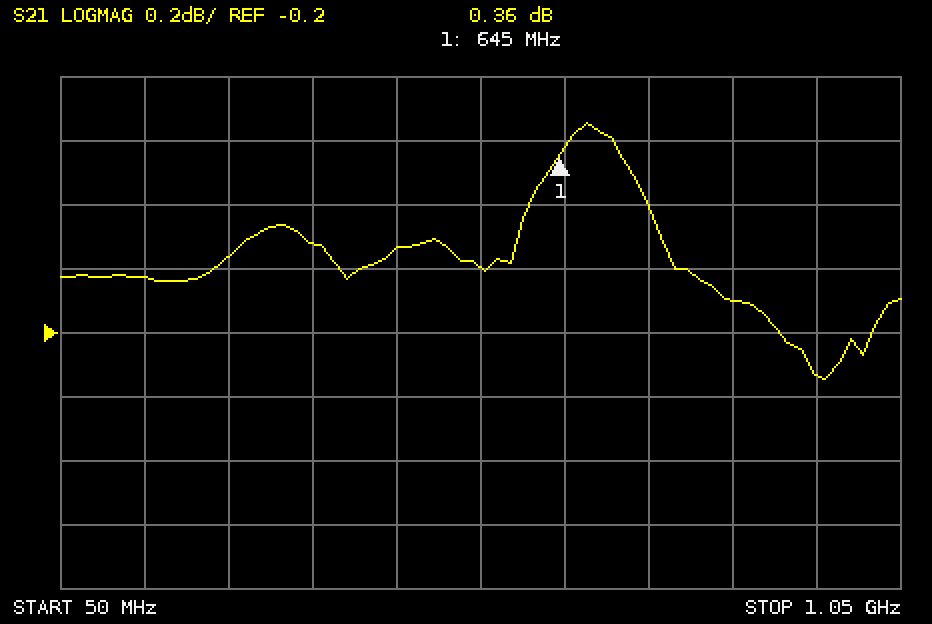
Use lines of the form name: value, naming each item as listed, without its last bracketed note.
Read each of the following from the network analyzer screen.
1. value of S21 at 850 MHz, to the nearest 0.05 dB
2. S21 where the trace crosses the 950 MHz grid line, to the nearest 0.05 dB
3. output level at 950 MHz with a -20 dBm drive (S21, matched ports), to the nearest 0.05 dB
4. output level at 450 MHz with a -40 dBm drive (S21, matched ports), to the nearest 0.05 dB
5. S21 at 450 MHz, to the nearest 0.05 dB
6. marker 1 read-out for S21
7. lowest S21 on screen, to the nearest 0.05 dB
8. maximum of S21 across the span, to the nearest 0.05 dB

value of S21 at 850 MHz, to the nearest 0.05 dB: -0.10 dB
S21 where the trace crosses the 950 MHz grid line, to the nearest 0.05 dB: -0.35 dB
output level at 950 MHz with a -20 dBm drive (S21, matched ports), to the nearest 0.05 dB: -20.35 dBm
output level at 450 MHz with a -40 dBm drive (S21, matched ports), to the nearest 0.05 dB: -39.95 dBm
S21 at 450 MHz, to the nearest 0.05 dB: 0.05 dB
marker 1 read-out for S21: 0.36 dB
lowest S21 on screen, to the nearest 0.05 dB: -0.35 dB
maximum of S21 across the span, to the nearest 0.05 dB: 0.45 dB
